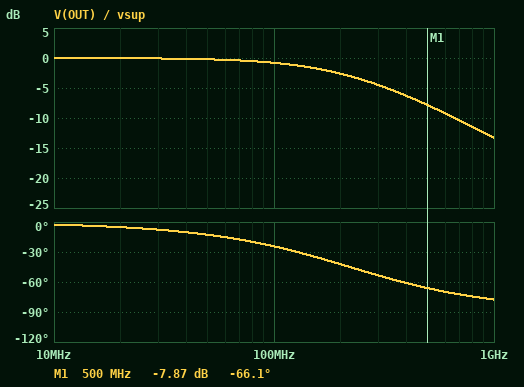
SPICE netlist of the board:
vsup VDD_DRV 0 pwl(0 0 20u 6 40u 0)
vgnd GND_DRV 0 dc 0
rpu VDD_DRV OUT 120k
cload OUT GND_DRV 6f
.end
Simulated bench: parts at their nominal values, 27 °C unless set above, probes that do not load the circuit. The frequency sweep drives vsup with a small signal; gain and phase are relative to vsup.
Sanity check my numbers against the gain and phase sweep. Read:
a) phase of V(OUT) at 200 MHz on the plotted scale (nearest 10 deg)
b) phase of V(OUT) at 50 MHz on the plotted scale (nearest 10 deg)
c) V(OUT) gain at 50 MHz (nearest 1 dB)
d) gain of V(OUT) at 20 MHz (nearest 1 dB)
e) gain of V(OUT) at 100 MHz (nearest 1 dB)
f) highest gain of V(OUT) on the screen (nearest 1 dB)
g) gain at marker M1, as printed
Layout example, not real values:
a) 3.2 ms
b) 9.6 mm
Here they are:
a) -40 deg
b) -10 deg
c) 0 dB
d) 0 dB
e) -1 dB
f) 0 dB
g) -7.87 dB
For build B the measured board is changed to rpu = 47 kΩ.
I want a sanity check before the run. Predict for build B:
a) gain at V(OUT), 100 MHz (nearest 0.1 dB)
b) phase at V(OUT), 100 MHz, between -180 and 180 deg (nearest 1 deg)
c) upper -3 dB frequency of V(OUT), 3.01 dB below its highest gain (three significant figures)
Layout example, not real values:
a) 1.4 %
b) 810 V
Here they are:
a) -0.1 dB
b) -10 deg
c) 564 MHz
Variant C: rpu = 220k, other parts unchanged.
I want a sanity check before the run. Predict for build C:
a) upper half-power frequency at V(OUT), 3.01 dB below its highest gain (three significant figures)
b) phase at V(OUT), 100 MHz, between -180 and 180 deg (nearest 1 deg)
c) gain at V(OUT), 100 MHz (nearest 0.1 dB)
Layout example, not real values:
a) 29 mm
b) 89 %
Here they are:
a) 121 MHz
b) -40 deg
c) -2.3 dB
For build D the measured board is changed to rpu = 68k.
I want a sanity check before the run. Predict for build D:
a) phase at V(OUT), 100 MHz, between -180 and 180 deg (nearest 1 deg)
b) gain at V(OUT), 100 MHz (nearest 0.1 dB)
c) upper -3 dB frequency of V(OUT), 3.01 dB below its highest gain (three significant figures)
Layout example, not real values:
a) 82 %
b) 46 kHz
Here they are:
a) -14 deg
b) -0.3 dB
c) 390 MHz
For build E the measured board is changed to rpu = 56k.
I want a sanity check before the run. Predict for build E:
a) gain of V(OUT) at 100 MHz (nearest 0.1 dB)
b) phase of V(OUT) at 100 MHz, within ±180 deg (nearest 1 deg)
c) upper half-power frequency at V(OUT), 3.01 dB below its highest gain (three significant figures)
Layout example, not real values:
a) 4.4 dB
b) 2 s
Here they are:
a) -0.2 dB
b) -12 deg
c) 474 MHz
